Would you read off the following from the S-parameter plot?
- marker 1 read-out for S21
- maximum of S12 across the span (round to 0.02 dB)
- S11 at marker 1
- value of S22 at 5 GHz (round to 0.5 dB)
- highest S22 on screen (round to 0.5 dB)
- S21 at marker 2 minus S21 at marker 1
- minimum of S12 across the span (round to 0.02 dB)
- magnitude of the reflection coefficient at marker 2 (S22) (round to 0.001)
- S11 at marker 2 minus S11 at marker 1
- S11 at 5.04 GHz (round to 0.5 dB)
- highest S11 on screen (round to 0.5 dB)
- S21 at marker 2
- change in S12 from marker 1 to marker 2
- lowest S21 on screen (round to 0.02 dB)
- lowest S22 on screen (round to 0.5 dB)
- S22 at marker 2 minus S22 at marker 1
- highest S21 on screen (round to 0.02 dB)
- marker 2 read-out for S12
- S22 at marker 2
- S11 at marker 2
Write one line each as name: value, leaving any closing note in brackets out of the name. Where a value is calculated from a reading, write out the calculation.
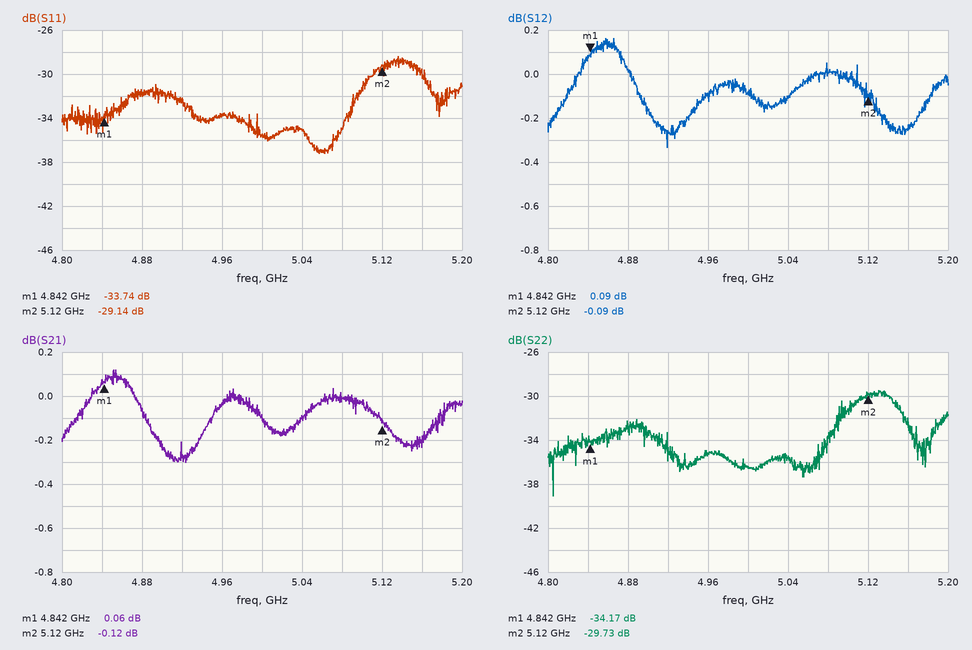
marker 1 read-out for S21: 0.06 dB
maximum of S12 across the span: 0.16 dB
S11 at marker 1: -33.74 dB
value of S22 at 5 GHz: -36.5 dB
highest S22 on screen: -29.5 dB
S21 at marker 2 minus S21 at marker 1: -0.12 − (0.06) = -0.18 dB
minimum of S12 across the span: -0.34 dB
magnitude of the reflection coefficient at marker 2 (S22): 10^(-29.73/20) ≈ 0.033
S11 at marker 2 minus S11 at marker 1: -29.14 − (-33.74) = 4.60 dB
S11 at 5.04 GHz: -35.0 dB
highest S11 on screen: -28.5 dB
S21 at marker 2: -0.12 dB
change in S12 from marker 1 to marker 2: -0.09 − (0.09) = -0.18 dB
lowest S21 on screen: -0.30 dB
lowest S22 on screen: -39.0 dB
S22 at marker 2 minus S22 at marker 1: -29.73 − (-34.17) = 4.44 dB
highest S21 on screen: 0.12 dB
marker 2 read-out for S12: -0.09 dB
S22 at marker 2: -29.73 dB
S11 at marker 2: -29.14 dB
